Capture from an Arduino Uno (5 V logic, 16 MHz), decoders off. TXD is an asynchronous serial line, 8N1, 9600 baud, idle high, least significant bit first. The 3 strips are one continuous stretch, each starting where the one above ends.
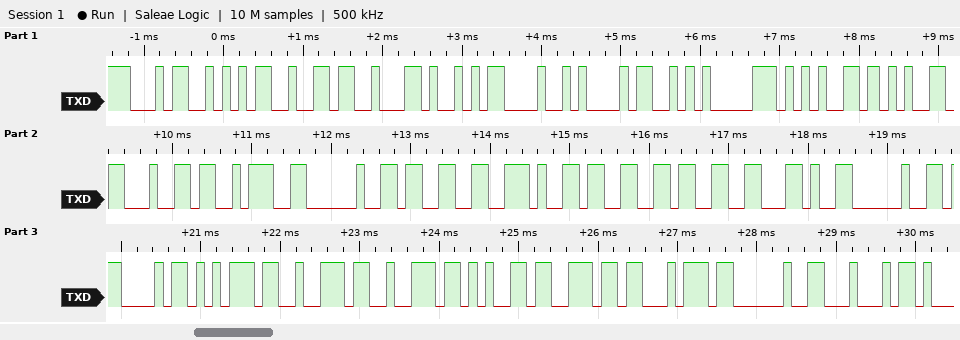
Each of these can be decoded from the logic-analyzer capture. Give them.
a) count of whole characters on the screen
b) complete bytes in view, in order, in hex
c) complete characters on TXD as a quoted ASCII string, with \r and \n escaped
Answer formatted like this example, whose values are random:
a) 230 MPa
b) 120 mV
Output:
a) 28
b) 34 35 36 2C 0D 0A 53 70 65 65 64 3A 20 33 2E 33 33 2C 20 43 75 72 72 65 6E 74 20 44
c) "456,\r\nSpeed: 3.33, Current D"
